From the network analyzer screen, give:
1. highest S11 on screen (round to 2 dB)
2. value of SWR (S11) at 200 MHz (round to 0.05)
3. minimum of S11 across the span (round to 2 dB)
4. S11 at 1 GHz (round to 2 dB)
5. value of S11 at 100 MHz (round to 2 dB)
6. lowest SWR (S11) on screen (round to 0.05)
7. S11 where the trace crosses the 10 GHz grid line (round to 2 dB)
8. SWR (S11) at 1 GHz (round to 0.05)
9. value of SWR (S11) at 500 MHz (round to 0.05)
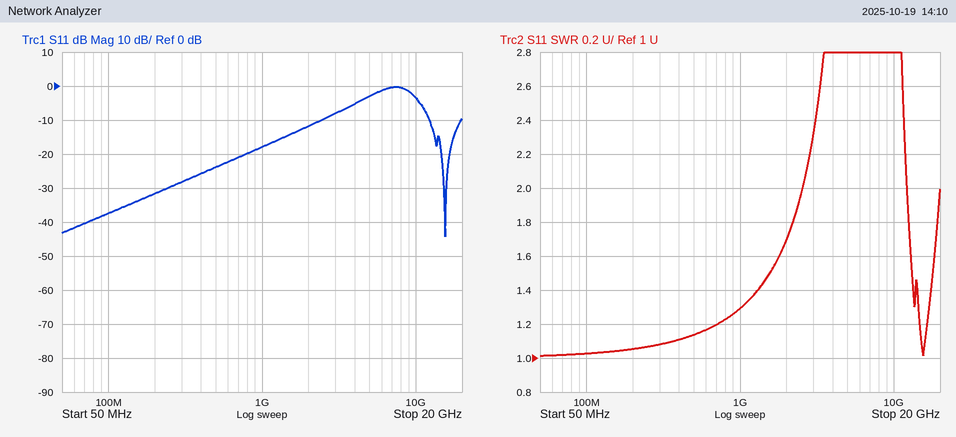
0 dB
1.05
-44 dB
-18 dB
-38 dB
1.00
-4 dB
1.30
1.15
